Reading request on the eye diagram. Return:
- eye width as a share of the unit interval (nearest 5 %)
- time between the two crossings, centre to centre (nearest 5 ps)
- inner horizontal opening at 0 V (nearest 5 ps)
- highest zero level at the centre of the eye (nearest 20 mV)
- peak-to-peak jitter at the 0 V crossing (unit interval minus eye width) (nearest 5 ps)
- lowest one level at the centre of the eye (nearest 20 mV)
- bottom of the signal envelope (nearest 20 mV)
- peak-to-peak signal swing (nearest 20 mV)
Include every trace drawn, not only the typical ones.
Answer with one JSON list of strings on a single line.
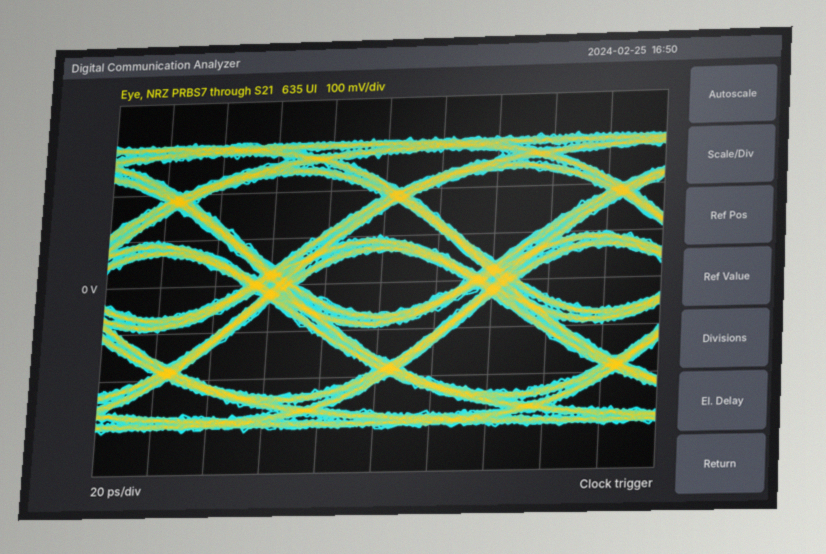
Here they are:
["75 %", "80 ps", "60 ps", "-60 mV", "20 ps", "60 mV", "-320 mV", "620 mV"]
